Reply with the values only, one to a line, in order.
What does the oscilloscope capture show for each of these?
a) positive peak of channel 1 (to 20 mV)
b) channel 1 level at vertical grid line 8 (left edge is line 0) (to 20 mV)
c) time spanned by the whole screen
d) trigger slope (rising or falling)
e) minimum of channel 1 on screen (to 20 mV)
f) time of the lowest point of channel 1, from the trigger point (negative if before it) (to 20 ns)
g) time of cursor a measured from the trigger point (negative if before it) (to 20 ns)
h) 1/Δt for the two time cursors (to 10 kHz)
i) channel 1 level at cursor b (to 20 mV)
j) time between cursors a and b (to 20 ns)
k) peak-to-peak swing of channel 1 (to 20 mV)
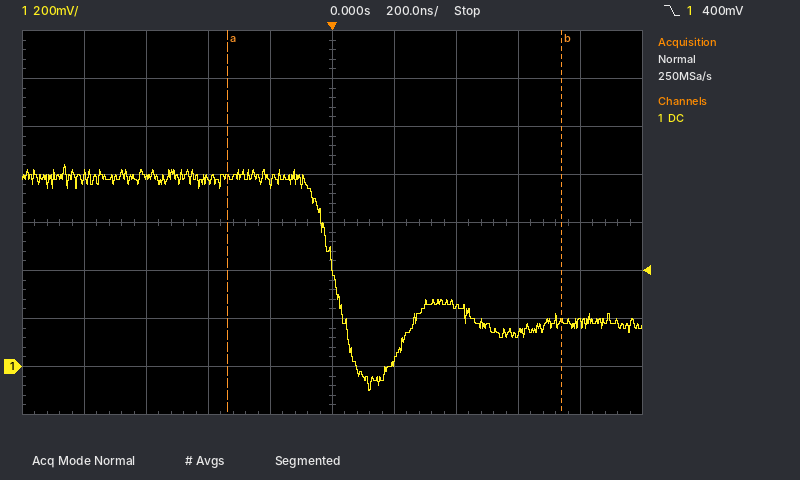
840 mV
140 mV
2 µs
falling
-100 mV
+120 ns
-340 ns
930 kHz
180 mV
1.08 µs
940 mV
